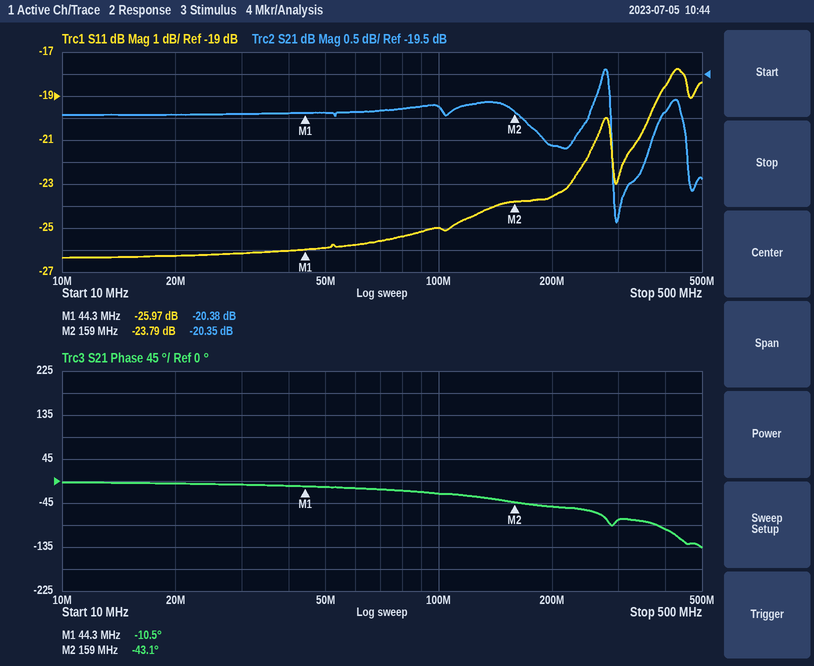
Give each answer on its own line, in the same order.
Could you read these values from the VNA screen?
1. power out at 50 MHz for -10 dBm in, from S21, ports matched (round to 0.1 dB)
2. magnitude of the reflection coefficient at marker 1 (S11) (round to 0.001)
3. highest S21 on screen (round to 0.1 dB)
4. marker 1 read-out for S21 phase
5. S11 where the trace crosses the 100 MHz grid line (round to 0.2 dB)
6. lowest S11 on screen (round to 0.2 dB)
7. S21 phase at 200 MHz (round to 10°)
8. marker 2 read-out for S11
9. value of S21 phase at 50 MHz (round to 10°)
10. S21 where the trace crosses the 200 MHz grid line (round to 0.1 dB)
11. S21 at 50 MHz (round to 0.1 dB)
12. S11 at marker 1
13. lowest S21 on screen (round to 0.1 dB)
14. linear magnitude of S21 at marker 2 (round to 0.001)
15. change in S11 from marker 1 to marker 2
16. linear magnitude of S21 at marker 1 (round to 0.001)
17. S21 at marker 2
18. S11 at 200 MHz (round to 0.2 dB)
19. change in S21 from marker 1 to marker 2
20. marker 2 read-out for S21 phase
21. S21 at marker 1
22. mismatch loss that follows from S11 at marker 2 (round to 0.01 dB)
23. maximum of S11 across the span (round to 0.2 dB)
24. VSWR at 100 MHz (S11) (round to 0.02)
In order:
-30.4 dBm
0.050
-19.4 dB
-10.5°
-25.0 dB
-26.4 dB
-50°
-23.79 dB
-10°
-21.1 dB
-20.4 dB
-25.97 dB
-22.9 dB
0.096
2.18 dB
0.096
-20.35 dB
-23.6 dB
0.03 dB
-43.1°
-20.38 dB
0.02 dB
-17.8 dB
1.12
